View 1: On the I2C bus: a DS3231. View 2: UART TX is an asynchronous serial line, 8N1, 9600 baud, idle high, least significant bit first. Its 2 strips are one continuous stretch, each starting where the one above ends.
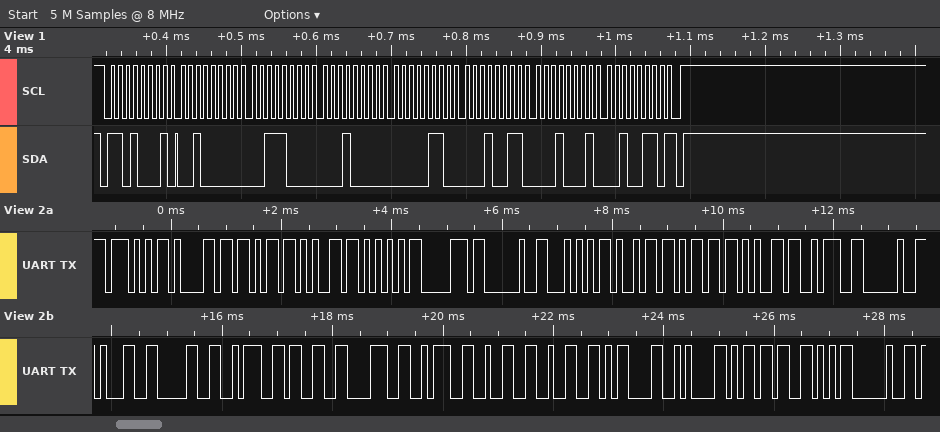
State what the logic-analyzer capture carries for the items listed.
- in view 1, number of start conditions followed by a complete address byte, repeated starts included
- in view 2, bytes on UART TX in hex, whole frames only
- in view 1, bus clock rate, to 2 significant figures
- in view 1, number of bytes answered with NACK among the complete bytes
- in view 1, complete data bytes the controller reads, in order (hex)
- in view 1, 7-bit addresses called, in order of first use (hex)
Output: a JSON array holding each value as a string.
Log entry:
["1", "57 61 6B 65 55 70 20 54 69 6D 65 3A 20 31 30 3A 33 38 3A 32 32 0D 0A 6D 56 20", "100 kHz", "1", "20 38 10 06 13 11 26", "0x68"]
